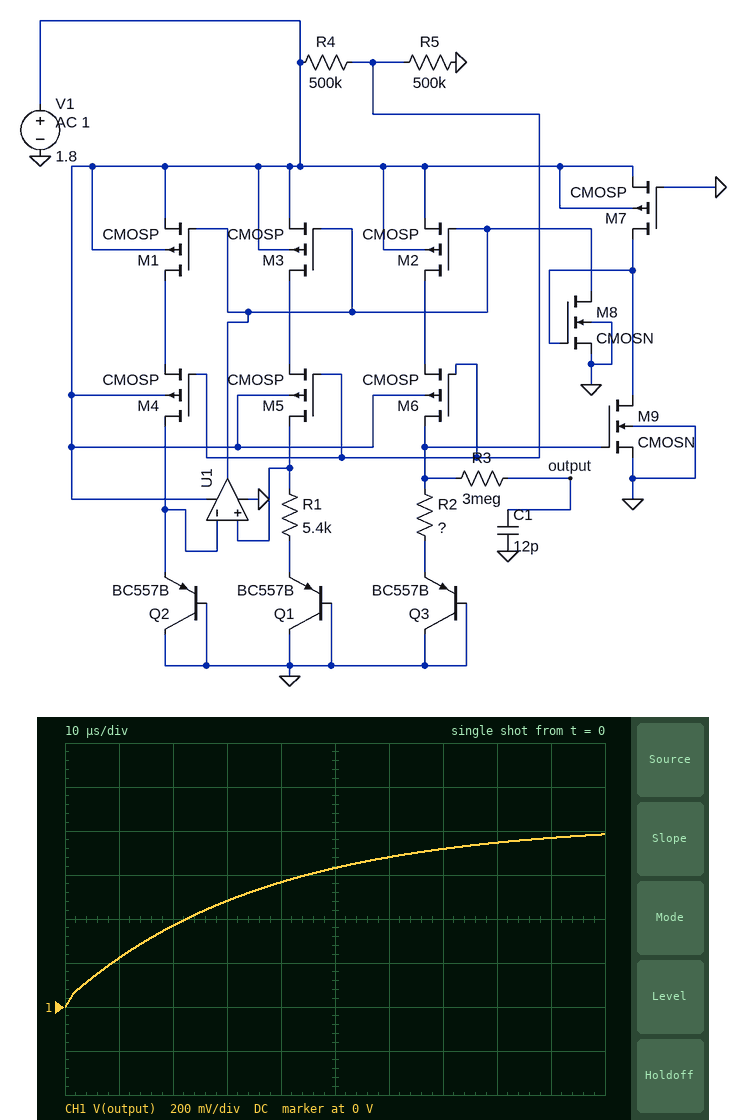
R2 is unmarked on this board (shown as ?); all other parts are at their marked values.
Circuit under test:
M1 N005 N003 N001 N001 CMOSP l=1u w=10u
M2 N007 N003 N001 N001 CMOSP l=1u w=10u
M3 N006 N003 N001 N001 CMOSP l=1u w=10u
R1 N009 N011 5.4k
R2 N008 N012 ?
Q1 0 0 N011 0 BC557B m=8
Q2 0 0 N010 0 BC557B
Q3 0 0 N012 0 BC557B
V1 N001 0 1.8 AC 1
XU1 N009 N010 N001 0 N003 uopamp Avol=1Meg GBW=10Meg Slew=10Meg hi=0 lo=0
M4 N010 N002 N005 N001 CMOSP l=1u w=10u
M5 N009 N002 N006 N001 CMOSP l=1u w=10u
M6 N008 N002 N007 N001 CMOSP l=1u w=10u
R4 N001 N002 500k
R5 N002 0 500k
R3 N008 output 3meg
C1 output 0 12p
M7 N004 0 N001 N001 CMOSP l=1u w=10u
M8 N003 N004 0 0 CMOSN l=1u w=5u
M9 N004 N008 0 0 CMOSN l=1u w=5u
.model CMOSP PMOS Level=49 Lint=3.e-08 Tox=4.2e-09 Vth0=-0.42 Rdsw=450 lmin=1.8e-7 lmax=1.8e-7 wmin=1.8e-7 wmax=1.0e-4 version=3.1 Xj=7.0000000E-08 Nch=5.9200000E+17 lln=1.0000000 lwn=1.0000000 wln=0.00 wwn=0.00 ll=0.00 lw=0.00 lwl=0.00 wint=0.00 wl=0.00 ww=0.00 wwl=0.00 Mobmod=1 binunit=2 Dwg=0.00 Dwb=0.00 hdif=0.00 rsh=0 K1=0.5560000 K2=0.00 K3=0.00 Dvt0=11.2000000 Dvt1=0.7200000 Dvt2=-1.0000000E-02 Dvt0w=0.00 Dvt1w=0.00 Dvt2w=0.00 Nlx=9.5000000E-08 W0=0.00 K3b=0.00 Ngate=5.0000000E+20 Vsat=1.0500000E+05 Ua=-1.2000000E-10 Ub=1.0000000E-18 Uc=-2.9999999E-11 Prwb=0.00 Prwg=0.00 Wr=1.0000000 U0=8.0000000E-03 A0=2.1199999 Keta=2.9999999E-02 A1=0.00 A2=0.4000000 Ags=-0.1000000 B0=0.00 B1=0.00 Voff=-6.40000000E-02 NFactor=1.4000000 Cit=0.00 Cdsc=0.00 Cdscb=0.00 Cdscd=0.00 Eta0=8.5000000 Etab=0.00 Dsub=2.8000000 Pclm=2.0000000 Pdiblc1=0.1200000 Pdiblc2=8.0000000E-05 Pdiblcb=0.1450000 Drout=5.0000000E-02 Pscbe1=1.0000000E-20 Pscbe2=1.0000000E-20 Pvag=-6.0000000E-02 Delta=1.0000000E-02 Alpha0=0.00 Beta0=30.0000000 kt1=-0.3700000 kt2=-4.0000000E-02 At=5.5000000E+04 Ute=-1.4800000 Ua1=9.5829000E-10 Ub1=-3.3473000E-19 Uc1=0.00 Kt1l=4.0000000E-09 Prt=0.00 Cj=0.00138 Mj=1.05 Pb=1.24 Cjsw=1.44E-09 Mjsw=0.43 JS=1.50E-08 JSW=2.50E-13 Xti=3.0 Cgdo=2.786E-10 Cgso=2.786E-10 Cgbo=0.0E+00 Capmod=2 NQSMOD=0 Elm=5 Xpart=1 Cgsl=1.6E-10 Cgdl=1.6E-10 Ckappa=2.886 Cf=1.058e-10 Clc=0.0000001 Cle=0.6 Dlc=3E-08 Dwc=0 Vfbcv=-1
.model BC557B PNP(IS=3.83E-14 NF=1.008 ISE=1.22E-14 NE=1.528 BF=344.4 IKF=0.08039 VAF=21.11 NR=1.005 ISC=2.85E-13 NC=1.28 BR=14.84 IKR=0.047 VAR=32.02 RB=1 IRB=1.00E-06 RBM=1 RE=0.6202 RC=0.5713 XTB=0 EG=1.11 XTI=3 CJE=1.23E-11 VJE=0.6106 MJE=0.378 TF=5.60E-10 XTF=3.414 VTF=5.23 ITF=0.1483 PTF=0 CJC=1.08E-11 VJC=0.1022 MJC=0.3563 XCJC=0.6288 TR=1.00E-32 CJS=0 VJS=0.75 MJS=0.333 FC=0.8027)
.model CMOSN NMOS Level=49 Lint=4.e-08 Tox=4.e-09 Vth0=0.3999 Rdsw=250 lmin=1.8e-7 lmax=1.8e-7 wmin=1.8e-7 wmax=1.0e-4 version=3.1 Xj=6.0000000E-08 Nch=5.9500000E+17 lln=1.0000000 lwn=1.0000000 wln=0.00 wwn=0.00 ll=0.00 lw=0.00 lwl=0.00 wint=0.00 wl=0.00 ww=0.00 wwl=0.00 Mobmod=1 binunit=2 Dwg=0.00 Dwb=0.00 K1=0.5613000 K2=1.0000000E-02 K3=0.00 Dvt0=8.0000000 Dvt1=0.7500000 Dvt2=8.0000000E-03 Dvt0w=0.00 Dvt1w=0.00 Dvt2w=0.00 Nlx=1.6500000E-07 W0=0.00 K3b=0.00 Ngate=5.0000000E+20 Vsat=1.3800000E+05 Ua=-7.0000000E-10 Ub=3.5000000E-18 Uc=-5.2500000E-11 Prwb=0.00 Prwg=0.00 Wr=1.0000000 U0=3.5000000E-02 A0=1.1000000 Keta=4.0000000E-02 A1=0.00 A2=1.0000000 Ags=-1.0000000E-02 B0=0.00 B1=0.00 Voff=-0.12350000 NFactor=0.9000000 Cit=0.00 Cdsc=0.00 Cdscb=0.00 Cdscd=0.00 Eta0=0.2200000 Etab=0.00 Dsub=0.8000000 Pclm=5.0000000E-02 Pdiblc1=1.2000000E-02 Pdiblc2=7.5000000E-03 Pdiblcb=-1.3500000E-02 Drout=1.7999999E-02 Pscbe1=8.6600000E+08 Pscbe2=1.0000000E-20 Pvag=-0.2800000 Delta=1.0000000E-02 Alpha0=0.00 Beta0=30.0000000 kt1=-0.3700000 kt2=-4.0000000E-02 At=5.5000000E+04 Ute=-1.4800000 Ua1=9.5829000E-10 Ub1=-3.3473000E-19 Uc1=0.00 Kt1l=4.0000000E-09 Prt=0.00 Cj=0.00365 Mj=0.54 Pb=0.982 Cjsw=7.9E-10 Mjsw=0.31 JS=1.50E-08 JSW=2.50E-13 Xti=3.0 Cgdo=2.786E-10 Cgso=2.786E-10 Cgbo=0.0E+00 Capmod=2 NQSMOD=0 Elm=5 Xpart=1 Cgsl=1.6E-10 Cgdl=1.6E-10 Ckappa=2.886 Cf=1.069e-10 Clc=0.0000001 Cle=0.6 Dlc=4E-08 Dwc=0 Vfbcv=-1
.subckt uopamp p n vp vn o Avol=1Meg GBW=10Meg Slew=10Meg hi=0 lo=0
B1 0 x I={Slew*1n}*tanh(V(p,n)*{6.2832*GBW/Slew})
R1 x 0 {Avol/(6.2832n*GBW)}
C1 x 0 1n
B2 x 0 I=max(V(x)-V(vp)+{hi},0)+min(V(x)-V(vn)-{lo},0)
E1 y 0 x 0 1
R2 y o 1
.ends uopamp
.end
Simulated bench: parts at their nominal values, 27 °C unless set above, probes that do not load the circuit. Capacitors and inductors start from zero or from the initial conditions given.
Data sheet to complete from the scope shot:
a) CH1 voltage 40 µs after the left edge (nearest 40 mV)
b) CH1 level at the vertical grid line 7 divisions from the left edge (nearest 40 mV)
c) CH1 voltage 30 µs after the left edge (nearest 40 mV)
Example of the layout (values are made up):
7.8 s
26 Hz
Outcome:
560 mV
720 mV
480 mV
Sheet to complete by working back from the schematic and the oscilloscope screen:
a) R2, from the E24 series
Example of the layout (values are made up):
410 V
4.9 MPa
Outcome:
33 kΩ
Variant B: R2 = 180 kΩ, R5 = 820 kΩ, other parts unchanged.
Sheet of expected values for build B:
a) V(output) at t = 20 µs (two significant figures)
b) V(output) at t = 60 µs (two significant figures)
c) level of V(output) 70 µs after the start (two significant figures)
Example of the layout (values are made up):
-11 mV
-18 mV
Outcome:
720 mV
1.4 V
1.5 V
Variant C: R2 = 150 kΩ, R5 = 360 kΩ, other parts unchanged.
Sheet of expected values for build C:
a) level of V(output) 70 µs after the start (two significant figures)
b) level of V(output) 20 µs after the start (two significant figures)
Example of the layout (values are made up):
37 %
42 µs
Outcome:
1.4 V
710 mV
